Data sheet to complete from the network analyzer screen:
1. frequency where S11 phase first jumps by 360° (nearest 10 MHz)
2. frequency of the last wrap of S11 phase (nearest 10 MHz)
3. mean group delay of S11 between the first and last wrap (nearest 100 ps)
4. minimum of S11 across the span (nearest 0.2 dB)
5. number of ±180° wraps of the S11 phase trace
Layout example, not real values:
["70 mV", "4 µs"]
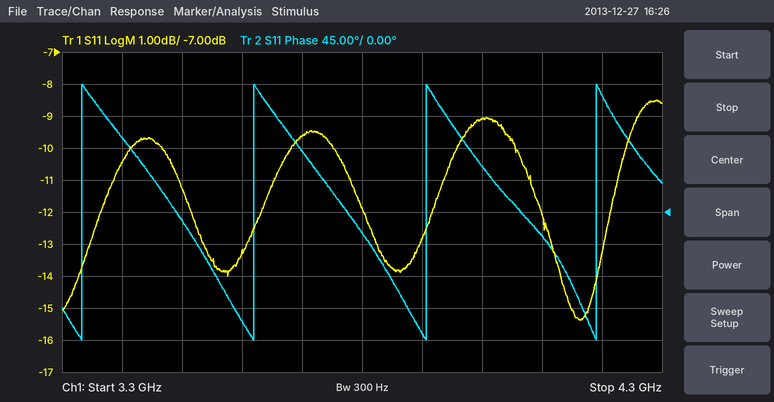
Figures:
["3.33 GHz", "4.19 GHz", "3.5 ns", "-15.4 dB", "4"]
